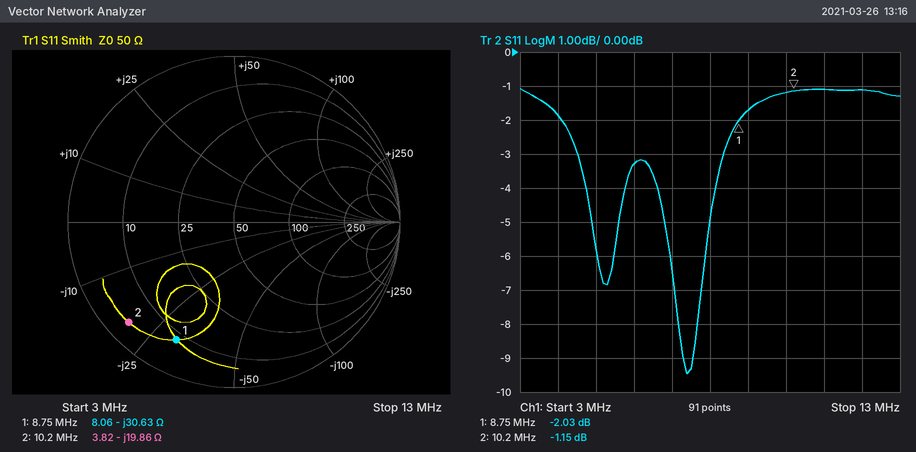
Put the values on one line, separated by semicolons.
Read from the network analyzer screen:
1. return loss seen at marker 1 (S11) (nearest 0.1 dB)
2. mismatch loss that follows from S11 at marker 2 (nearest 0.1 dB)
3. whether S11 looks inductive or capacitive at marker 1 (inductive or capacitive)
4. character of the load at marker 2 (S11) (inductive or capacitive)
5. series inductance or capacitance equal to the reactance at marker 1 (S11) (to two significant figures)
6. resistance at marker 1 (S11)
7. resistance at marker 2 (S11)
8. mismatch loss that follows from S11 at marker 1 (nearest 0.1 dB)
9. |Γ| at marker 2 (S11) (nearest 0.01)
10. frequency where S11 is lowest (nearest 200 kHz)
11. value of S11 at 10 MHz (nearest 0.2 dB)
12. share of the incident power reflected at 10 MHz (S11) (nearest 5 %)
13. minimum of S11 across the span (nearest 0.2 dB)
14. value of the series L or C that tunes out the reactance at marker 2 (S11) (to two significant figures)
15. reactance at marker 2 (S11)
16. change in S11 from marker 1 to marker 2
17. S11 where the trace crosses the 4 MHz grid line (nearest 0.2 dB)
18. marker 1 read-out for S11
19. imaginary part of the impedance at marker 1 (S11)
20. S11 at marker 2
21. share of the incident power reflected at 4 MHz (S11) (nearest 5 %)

2.0 dB; 6.3 dB; capacitive; capacitive; 590 pF; 8.06 Ω; 3.82 Ω; 4.3 dB; 0.88; 7.4 MHz; -1.2 dB; 75 %; -9.4 dB; 310 nH; -19.86 Ω; 0.88 dB; -1.8 dB; -2.03 dB; -30.63 Ω; -1.15 dB; 65 %
